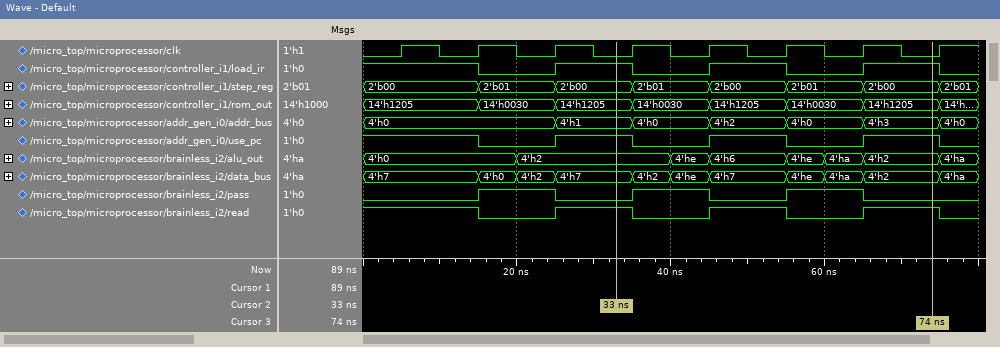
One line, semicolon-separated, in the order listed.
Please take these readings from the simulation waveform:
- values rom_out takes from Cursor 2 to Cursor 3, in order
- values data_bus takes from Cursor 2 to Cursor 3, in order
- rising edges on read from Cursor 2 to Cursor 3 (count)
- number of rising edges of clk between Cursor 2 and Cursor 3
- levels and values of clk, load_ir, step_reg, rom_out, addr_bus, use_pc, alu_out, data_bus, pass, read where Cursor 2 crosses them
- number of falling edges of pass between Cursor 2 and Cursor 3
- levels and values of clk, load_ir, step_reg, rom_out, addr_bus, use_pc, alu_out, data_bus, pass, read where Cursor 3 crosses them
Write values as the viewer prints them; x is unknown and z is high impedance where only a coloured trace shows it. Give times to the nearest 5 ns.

14'h1205, 14'h0030, 14'h1205, 14'h0030, 14'h1205; 4'h7, 4'h2, 4'he, 4'h7, 4'he, 4'ha, 4'h2; 2; 4; clk=0, load_ir=1, step_reg=2'b00, rom_out=14'h1205, addr_bus=4'h1, use_pc=1, alu_out=4'h2, data_bus=4'h7, pass=0, read=1; 2; clk=0, load_ir=1, step_reg=2'b00, rom_out=14'h1205, addr_bus=4'h3, use_pc=1, alu_out=4'h2, data_bus=4'h2, pass=0, read=1
